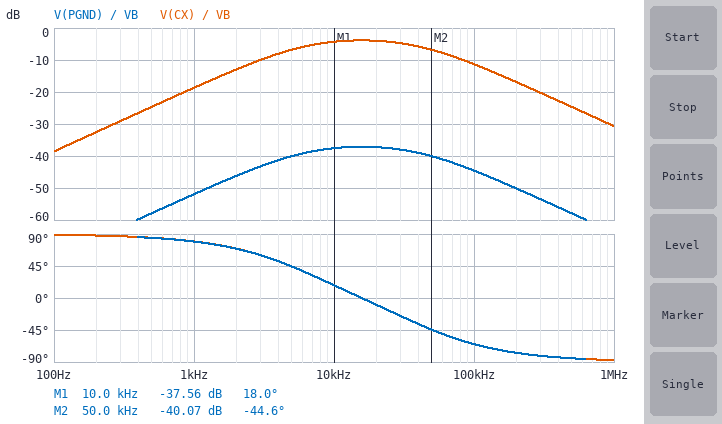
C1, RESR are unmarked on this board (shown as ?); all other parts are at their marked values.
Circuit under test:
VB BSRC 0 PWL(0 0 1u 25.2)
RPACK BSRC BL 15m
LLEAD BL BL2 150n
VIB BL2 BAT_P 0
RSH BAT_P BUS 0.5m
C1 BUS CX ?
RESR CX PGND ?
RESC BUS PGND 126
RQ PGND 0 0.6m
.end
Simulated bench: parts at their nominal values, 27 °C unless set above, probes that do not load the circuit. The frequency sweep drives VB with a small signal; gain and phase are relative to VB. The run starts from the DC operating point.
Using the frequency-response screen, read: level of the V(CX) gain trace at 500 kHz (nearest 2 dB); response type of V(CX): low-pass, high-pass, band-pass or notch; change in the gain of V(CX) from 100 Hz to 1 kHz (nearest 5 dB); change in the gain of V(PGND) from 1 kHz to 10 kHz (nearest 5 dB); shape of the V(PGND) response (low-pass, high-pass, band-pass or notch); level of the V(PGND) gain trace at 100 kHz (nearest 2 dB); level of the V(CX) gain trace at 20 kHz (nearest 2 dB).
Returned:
-24 dB
band-pass
20 dB
15 dB
band-pass
-44 dB
-4 dB
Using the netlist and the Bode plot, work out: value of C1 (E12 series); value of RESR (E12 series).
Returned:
680 µF
0.027 Ω
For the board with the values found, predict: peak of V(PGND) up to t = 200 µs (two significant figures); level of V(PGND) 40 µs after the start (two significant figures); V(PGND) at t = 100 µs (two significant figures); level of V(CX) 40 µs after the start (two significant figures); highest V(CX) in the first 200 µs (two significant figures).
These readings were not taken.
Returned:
290 mV
100 mV
9.6 mV
4.7 V
13 V
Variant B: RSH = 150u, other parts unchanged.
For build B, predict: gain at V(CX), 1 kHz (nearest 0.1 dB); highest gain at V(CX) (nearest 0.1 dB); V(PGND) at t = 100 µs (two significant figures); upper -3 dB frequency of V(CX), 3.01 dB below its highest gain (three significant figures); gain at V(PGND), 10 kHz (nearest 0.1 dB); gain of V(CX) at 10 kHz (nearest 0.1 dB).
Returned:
-18.7 dB
-3.8 dB
9.3 mV
50.3 kHz
-37.5 dB
-4.2 dB
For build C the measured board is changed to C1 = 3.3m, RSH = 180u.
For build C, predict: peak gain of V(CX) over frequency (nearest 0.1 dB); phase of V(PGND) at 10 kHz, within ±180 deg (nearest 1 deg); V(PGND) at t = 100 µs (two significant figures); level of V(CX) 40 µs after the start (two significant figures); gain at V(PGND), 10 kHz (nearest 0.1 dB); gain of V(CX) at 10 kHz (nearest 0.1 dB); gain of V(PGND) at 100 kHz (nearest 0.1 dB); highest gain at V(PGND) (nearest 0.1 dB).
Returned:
-3.8 dB
-6 deg
180 mV
13 V
-37.1 dB
-3.9 dB
-44.7 dB
-37.1 dB
